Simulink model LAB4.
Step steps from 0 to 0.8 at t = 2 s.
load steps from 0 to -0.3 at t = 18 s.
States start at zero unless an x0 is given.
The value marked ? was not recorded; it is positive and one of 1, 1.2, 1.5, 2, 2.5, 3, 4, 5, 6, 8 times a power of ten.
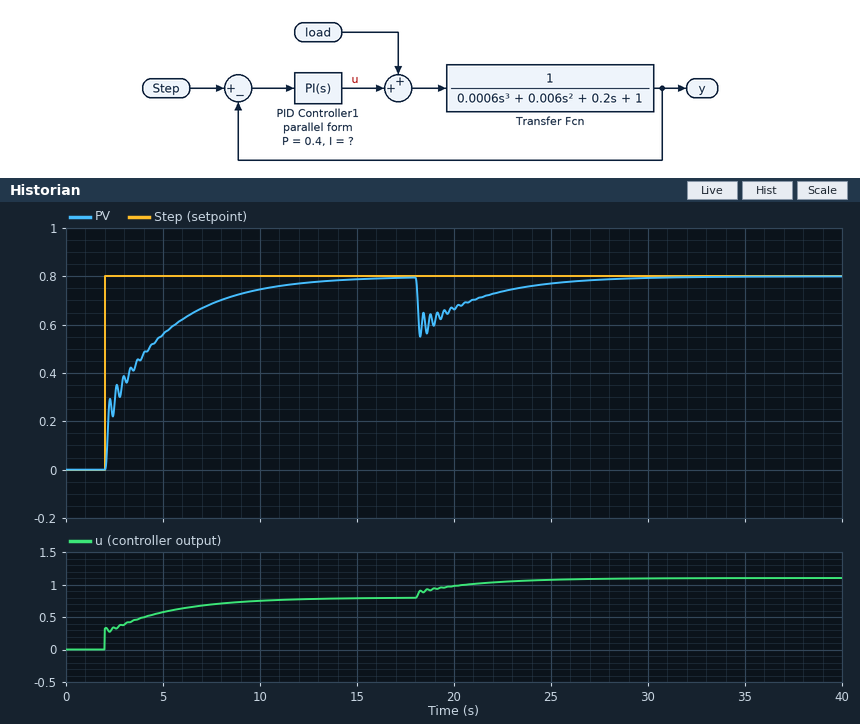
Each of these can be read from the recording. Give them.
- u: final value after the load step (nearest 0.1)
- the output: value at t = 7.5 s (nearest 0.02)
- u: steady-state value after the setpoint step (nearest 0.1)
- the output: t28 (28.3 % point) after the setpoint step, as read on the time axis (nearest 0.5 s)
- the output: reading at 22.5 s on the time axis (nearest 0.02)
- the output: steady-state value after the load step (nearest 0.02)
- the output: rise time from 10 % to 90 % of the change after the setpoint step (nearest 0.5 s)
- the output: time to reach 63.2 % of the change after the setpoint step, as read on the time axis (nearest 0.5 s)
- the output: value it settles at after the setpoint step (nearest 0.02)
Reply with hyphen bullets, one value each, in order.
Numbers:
- 1.1
- 0.68
- 0.8
- 2.0 s
- 0.74
- 0.80
- 6.5 s
- 4.5 s
- 0.80
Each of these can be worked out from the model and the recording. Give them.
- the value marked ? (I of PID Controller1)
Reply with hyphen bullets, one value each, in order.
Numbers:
- 0.4
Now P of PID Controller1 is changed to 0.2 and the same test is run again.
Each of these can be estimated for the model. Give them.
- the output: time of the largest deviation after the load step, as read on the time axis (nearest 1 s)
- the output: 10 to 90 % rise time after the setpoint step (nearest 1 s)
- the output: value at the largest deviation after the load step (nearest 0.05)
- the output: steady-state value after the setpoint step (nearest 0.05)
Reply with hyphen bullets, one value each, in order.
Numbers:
- 18 s
- 6 s
- 0.55
- 0.80
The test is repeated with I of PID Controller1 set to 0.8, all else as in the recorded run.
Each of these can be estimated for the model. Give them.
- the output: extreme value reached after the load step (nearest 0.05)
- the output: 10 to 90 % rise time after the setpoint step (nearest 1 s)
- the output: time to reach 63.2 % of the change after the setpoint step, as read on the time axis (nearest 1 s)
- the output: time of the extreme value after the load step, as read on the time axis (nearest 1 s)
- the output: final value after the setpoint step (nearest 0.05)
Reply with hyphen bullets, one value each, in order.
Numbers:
- 0.55
- 3 s
- 3 s
- 18 s
- 0.80
